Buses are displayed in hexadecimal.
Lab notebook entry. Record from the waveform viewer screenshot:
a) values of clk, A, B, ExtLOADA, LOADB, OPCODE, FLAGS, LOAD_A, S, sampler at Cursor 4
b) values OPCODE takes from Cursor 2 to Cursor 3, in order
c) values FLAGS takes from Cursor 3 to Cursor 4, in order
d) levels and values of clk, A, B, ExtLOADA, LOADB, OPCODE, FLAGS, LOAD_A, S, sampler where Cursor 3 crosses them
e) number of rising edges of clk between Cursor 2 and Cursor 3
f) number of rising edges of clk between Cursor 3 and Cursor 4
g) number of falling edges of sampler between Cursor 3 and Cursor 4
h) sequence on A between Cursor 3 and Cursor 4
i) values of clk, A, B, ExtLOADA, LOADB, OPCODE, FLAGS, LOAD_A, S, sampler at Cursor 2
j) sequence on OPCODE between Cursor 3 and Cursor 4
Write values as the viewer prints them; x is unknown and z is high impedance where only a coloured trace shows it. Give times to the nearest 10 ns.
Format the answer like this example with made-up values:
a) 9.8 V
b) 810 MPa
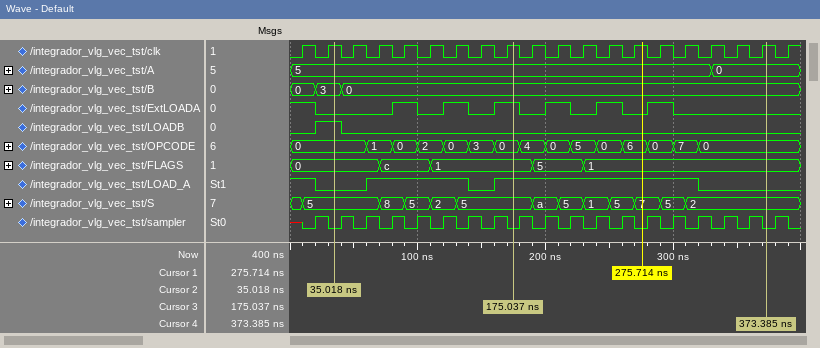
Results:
a) clk=1, A=0, B=0, ExtLOADA=0, LOADB=0, OPCODE=0, FLAGS=1, LOAD_A=0, S=2, sampler=0
b) 0, 1, 0, 2, 0, 3, 0
c) 1, 5, 1
d) clk=1, A=5, B=0, ExtLOADA=1, LOADB=0, OPCODE=0, FLAGS=1, LOAD_A=1, S=5, sampler=0
e) 7
f) 10
g) 10
h) 5, 0
i) clk=1, A=5, B=3, ExtLOADA=0, LOADB=1, OPCODE=0, FLAGS=0, LOAD_A=0, S=5, sampler=0
j) 0, 4, 0, 5, 0, 6, 0, 7, 0
